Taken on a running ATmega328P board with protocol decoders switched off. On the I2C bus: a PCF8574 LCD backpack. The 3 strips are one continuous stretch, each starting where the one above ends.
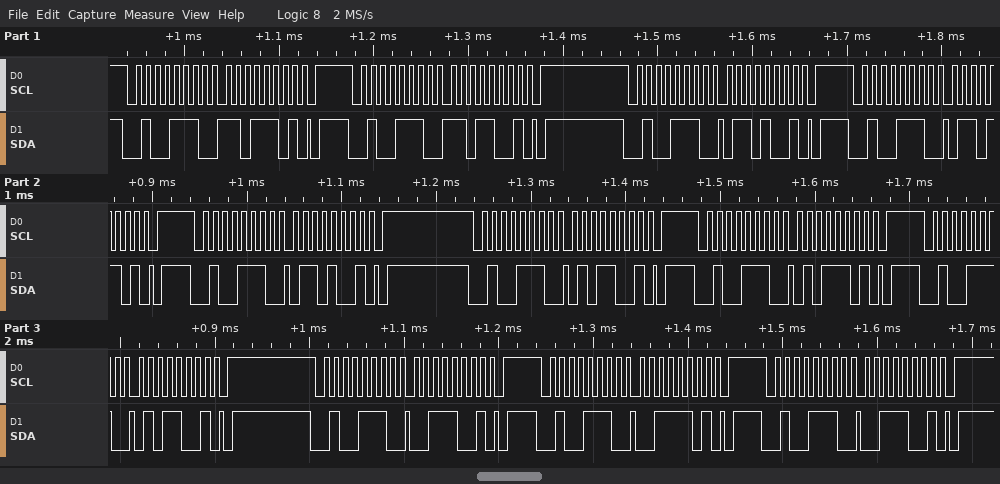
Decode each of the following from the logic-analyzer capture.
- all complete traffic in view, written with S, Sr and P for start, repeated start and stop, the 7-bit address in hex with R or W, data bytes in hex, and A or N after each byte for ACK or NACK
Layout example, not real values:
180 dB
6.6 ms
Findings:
S 27W A DD A P S 27W A D9 A P S 27W A 69 A P S 27W A 6D A P S 27W A 69 A P S 27W A 59 A P S 27W A 5D A P S 27W A 59 A P S 27W A 39 A P S 27W A 3D A P S 27W A 39 A P
